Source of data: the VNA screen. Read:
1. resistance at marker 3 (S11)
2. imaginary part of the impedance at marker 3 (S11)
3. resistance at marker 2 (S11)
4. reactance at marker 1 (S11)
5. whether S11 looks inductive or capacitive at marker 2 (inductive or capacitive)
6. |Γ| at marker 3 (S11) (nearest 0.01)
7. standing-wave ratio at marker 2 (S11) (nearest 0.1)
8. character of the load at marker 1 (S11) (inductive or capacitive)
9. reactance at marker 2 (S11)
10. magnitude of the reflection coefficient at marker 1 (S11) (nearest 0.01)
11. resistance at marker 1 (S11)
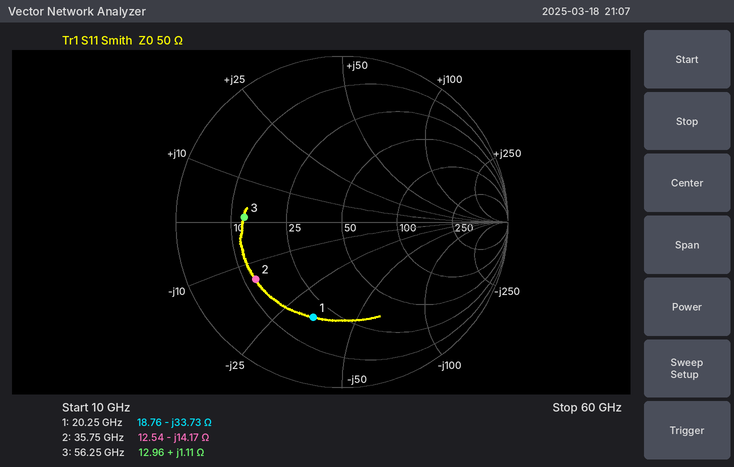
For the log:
12.96 Ω
+1.11 Ω
12.54 Ω
-33.73 Ω
capacitive
0.59
4.3
capacitive
-14.17 Ω
0.60
18.76 Ω
